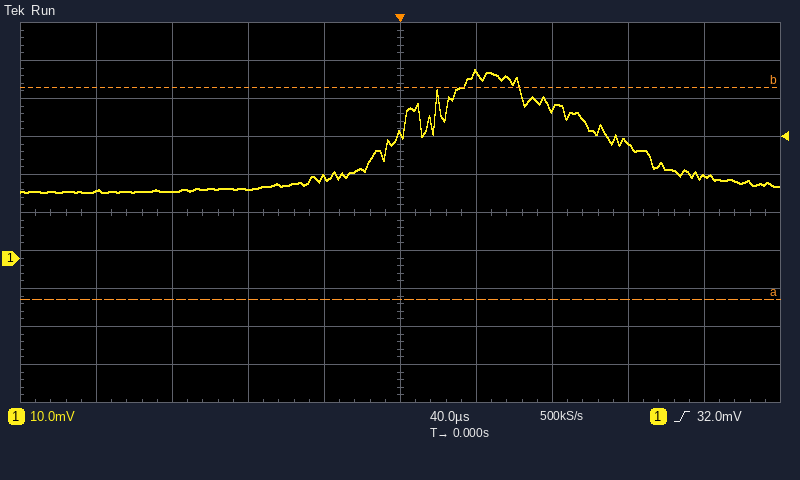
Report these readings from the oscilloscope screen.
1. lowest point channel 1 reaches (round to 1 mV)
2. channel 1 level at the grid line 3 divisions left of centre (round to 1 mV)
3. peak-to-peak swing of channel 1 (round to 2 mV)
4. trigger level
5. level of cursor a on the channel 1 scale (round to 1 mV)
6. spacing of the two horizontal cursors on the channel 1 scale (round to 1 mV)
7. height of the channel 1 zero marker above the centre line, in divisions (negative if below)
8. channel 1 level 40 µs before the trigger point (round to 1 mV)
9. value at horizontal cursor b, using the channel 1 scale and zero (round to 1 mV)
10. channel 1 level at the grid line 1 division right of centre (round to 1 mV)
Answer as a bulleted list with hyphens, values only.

- 17 mV
- 18 mV
- 32 mV
- 32.0 mV
- -11 mV
- 56 mV
- -1.2 div
- 21 mV
- 45 mV
- 49 mV
